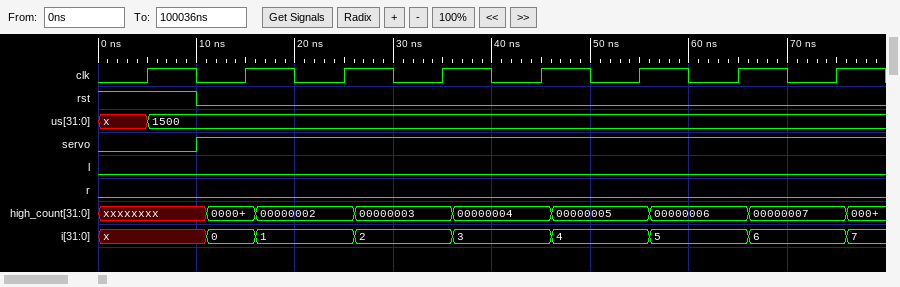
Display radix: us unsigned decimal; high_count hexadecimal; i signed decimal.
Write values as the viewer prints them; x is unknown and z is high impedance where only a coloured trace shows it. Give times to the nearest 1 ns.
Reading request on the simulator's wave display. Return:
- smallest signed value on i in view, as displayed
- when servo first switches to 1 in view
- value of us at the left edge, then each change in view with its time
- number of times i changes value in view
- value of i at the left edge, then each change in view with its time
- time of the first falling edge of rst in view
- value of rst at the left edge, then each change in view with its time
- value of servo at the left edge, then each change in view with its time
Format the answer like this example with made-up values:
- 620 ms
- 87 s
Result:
- 0
- 10 ns
- x, 1500 at 5 ns
- 8
- x, 0 at 11 ns, 1 at 16 ns, 2 at 26 ns, 3 at 36 ns, 4 at 46 ns, 5 at 56 ns, 6 at 66 ns, 7 at 76 ns
- 10 ns
- 1, 0 at 10 ns
- 0, 1 at 10 ns
